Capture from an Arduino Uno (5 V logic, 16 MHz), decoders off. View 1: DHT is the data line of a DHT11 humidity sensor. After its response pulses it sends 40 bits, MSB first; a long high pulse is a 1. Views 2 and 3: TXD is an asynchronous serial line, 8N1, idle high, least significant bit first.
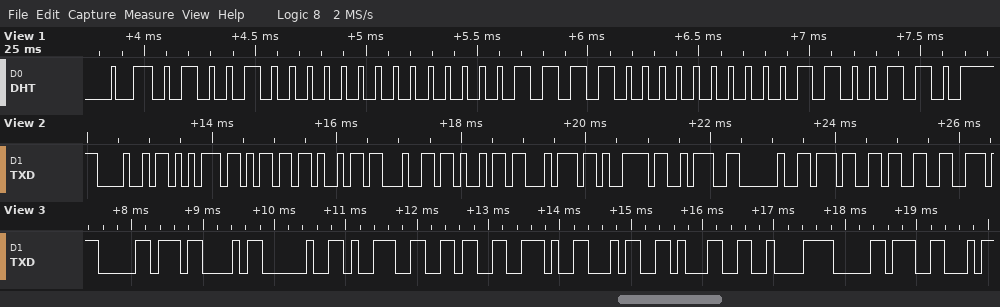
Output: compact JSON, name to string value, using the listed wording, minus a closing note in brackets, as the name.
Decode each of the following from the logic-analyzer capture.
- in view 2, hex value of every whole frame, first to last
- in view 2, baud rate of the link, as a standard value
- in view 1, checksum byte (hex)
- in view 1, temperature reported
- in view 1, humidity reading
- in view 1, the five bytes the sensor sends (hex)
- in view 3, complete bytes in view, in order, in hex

{"in view 2, hex value of every whole frame, first to last": "48 75 6D 69 64 69 74 79 3A 20 37 33", "in view 2, baud rate of the link, as a standard value": "9600 baud", "in view 1, checksum byte": "0x66", "in view 1, temperature reported": "30.0 °C", "in view 1, humidity reading": "72 %", "in view 1, the five bytes the sensor sends": "48 00 1E 00 66", "in view 3, complete bytes in view, in order, in hex": "B0 43 20 39 36 2E 34 31 C2 B0 46"}
